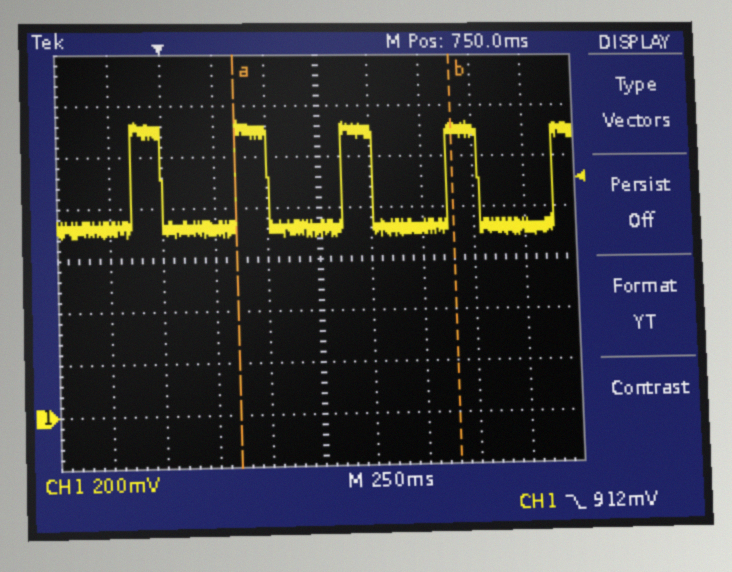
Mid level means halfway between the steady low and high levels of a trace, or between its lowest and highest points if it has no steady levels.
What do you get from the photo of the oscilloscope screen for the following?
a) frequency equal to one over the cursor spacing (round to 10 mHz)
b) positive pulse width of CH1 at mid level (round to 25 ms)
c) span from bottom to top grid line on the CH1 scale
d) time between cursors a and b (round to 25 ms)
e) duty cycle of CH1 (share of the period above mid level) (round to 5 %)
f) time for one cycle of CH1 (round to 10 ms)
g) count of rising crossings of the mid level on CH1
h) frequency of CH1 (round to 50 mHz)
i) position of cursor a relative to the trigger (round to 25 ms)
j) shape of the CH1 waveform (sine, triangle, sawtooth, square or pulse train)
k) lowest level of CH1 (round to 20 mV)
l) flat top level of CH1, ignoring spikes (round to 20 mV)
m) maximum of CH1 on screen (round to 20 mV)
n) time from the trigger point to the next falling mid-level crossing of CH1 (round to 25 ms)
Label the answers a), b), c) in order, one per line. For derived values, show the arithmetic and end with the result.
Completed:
a) 1 / 1.050 s ≈ 950 mHz
b) 150 ms
c) 1.6 V
d) 1.050 s
e) 150 ms / 510 ms ≈ 29.4 %, so 30 % to the nearest 5 %
f) 510 ms
g) 5
h) 1 / 510 ms ≈ 1.96 Hz, so 1.95 Hz to the nearest 50 mHz
i) +350 ms
j) pulse train
k) 680 mV
l) 1.10 V
m) 1.14 V
n) 500 ms
